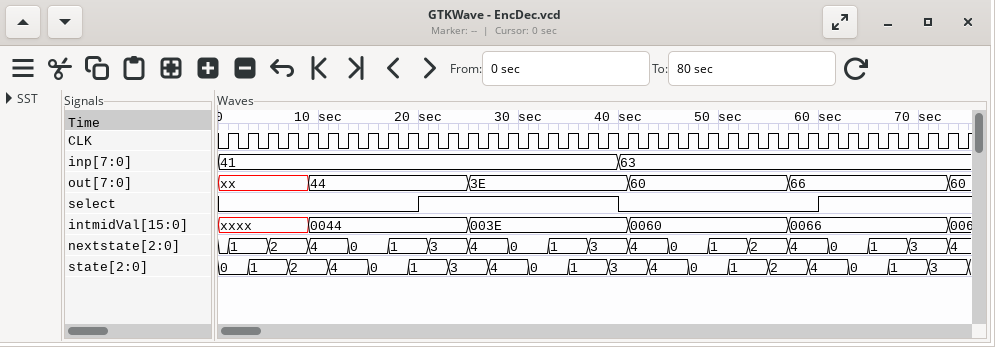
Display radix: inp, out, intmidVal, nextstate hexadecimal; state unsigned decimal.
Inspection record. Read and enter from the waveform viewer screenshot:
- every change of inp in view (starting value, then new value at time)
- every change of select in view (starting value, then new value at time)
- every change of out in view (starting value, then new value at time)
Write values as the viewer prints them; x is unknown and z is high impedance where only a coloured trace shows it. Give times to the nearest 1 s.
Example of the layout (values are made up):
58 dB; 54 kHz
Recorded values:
41, 63 at 40 s; 0, 1 at 20 s, 0 at 40 s, 1 at 60 s; xx, 44 at 9 s, 3E at 25 s, 60 at 41 s, 66 at 57 s, 60 at 73 s
